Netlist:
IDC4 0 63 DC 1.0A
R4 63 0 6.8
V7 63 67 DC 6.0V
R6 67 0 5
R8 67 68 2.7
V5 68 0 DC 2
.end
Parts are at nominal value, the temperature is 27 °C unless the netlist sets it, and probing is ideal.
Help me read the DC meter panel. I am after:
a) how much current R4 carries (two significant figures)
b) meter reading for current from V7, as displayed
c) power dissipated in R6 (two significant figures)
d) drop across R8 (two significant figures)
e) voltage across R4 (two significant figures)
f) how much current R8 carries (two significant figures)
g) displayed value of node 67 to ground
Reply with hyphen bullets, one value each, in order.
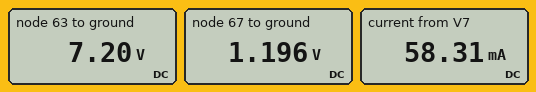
- 1.1 A
- 58.31 mA
- 290 mW
- 800 mV
- 7.2 V
- 300 mA
- 1.196 V
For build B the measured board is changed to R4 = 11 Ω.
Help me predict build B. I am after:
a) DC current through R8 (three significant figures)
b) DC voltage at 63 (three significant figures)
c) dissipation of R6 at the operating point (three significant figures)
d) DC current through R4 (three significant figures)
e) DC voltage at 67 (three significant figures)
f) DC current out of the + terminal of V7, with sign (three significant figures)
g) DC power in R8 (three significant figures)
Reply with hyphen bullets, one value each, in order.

- 71.3 mA
- 7.81 V
- 653 mW
- 710 mA
- 1.81 V
- -290 mA
- 13.7 mW
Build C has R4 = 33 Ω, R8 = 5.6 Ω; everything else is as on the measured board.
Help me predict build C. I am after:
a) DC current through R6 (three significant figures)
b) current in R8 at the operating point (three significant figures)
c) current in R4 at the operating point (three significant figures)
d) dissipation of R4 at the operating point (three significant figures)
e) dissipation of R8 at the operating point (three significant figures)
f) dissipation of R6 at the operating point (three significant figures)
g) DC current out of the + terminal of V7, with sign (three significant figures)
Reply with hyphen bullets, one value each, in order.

- 575 mA
- 156 mA
- 269 mA
- 2.39 W
- 137 mW
- 1.65 W
- -731 mA
